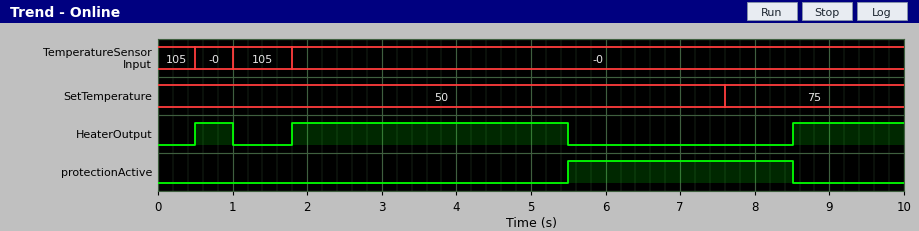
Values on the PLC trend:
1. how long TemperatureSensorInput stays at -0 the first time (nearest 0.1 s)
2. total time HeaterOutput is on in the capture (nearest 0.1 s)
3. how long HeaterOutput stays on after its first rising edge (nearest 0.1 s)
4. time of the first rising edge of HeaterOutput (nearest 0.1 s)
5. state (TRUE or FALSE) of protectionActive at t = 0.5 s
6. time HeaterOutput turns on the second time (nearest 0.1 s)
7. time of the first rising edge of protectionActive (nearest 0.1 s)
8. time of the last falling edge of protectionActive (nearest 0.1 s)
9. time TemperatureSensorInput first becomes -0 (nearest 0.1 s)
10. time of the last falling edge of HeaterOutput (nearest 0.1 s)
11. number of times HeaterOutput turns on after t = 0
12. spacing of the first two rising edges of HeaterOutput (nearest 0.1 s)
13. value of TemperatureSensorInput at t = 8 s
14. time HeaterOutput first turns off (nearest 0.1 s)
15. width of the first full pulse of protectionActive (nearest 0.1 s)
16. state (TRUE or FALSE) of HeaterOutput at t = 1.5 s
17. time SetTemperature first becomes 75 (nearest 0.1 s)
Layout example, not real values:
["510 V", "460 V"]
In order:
["0.5 s", "5.7 s", "0.5 s", "0.5 s", "FALSE", "1.8 s", "5.5 s", "8.5 s", "0.5 s", "5.5 s", "3", "1.3 s", "-0", "1.0 s", "3.0 s", "FALSE", "7.6 s"]
